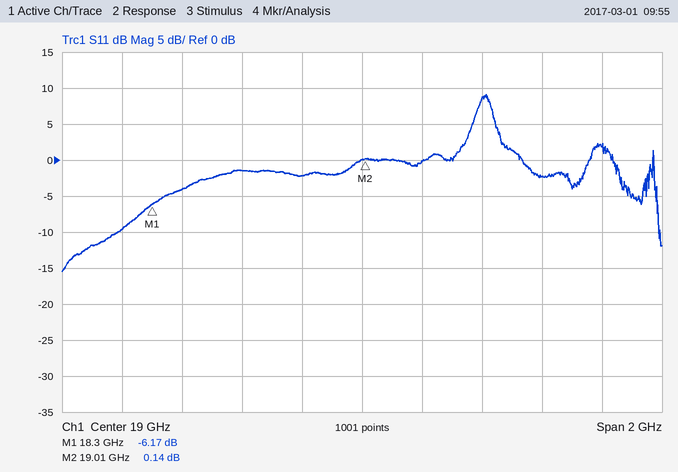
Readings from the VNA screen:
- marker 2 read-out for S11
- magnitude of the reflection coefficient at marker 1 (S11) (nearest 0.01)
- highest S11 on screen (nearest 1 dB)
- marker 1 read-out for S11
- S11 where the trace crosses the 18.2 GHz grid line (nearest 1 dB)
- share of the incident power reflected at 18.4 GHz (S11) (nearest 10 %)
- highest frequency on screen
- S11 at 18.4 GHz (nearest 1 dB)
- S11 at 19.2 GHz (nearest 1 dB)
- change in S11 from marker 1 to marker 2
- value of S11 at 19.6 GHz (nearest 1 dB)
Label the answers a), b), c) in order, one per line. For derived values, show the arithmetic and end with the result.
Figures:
a) 0.14 dB
b) 10^(-6.17/20) ≈ 0.49
c) 9 dB
d) -6.17 dB
e) -10 dB
f) 10^(-4/10) ≈ 40 %
g) 20 GHz
h) -4 dB
i) 0 dB
j) 0.14 − (-6.17) = 6.31 dB
k) -2 dB
